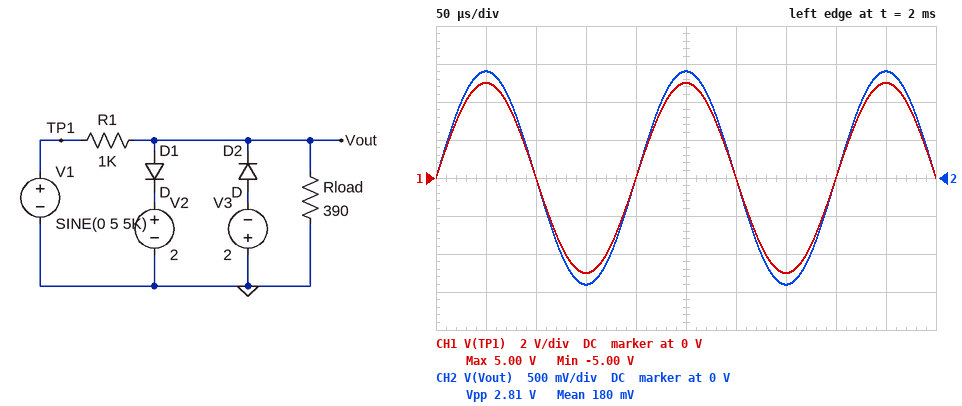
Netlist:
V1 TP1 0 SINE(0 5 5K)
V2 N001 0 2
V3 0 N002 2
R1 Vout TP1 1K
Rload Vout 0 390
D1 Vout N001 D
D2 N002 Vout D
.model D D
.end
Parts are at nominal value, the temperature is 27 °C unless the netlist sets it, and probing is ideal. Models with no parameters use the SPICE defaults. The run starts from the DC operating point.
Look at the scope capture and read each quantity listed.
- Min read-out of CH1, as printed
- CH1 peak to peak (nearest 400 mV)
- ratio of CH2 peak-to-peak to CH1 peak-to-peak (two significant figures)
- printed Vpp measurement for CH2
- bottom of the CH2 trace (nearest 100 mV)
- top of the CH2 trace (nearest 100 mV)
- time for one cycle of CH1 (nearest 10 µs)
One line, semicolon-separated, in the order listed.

-5.00 V; 10.0 V; 0.28; 2.81 V; -1.4 V; 1.4 V; 200 µs
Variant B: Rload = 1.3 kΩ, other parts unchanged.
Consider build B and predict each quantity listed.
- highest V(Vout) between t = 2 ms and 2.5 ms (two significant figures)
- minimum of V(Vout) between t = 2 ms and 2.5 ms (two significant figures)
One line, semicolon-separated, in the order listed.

2.6 V; -2.6 V
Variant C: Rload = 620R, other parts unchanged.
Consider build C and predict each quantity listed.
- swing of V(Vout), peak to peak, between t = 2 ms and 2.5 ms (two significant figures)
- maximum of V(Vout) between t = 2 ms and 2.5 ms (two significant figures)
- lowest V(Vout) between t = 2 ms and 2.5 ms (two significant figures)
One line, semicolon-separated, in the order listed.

3.8 V; 1.9 V; -1.9 V
